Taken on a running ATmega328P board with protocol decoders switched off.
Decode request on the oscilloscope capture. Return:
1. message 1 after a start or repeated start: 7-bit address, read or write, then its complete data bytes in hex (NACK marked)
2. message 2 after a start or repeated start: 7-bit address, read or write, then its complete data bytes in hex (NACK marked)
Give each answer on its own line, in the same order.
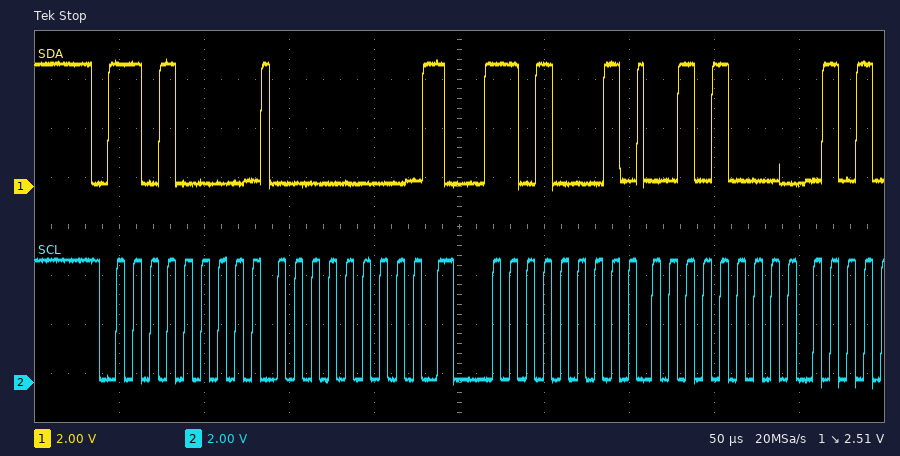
0x68 write: 00
0x68 read: 28
